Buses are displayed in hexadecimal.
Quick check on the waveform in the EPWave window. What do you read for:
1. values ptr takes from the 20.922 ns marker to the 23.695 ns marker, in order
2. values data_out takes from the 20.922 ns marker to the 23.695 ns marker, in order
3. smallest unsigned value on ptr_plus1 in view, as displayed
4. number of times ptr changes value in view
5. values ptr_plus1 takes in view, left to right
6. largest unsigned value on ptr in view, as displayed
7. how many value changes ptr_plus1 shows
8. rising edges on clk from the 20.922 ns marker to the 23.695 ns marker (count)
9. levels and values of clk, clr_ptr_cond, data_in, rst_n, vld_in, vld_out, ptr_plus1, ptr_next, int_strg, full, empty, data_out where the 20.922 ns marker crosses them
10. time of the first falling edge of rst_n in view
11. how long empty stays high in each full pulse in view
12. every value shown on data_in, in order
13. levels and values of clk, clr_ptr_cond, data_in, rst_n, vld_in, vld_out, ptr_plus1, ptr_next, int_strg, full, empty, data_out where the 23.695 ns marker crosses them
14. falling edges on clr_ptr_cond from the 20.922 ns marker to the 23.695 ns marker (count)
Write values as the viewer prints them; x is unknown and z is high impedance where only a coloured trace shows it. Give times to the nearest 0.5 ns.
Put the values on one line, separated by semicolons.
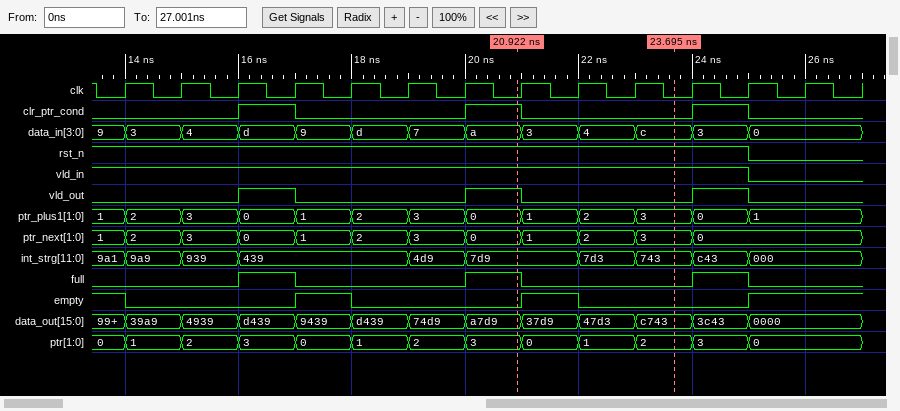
3, 0, 1, 2; a7d9, 37d9, 47d3, c743; 0; 12; 1, 2, 3, 0, 1, 2, 3, 0, 1, 2, 3, 0, 1; 3; 12; 3; clk=0, clr_ptr_cond=1, data_in=a, rst_n=1, vld_in=1, vld_out=1, ptr_plus1=0, ptr_next=0, int_strg=7d9, full=1, empty=0, data_out=a7d9; 25 ns; 1 ns, 1 ns; 9, 3, 4, d, 9, d, 7, a, 3, 4, c, 3, 0; clk=0, clr_ptr_cond=0, data_in=c, rst_n=1, vld_in=1, vld_out=0, ptr_plus1=3, ptr_next=3, int_strg=743, full=0, empty=0, data_out=c743; 1
